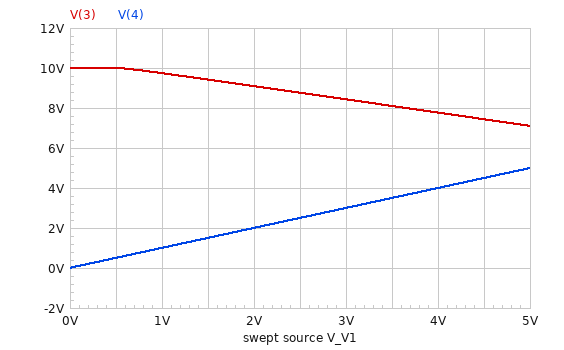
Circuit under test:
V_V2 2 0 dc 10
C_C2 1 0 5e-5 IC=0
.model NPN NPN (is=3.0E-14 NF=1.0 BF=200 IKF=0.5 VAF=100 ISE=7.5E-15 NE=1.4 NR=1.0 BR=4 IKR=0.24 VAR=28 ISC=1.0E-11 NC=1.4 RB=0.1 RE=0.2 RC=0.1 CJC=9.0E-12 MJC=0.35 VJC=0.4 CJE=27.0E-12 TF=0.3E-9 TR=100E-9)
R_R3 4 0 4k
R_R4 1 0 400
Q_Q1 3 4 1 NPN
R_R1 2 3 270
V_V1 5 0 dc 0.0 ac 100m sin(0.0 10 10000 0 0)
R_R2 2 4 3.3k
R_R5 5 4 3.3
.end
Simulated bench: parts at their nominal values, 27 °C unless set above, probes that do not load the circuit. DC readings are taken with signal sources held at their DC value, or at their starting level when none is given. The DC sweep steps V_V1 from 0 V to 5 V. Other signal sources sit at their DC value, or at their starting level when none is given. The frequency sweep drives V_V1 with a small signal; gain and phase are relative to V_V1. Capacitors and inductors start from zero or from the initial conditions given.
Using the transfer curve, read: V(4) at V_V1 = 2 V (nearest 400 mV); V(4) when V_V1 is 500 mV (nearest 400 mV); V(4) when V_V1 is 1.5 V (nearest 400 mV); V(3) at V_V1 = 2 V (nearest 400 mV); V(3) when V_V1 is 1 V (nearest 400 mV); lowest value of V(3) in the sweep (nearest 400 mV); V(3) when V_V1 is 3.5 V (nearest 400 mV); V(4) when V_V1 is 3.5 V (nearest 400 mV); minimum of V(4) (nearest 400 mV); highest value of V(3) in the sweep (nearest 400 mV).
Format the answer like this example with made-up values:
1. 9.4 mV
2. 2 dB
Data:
1. 2.0 V
2. 400 mV
3. 1.6 V
4. 9.2 V
5. 9.6 V
6. 7.2 V
7. 8.0 V
8. 3.6 V
9. 0 V
10. 10.0 V
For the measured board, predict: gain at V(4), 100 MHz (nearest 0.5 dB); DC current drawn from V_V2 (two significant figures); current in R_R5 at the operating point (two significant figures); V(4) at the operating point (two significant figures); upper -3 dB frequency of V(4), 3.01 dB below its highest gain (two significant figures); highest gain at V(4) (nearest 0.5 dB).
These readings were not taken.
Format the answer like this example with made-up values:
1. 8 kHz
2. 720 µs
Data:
1. 0 dB
2. 3.0 mA
3. 3.0 mA
4. 10 mV
5. 1.6 GHz
6. 0 dB
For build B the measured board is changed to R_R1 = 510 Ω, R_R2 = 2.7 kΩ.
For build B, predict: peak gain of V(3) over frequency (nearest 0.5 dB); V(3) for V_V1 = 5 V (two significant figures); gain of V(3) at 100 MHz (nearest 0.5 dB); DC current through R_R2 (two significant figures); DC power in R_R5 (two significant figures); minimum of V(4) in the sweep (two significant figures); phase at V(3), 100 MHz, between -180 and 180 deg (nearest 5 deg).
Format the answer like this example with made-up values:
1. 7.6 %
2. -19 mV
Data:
1. -0.5 dB
2. 4.5 V
3. -3.5 dB
4. 3.7 mA
5. 45 µW
6. 12 mV
7. 45 deg
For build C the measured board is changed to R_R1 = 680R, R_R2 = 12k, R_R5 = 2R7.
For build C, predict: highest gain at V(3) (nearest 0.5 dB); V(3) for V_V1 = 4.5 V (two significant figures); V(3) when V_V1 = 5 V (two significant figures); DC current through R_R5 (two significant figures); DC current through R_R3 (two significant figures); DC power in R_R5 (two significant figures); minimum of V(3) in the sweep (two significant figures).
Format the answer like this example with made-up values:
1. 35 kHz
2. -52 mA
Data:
1. -0.5 dB
2. 3.9 V
3. 4.3 V
4. 830 µA
5. 560 nA
6. 1.9 µW
7. 3.8 V
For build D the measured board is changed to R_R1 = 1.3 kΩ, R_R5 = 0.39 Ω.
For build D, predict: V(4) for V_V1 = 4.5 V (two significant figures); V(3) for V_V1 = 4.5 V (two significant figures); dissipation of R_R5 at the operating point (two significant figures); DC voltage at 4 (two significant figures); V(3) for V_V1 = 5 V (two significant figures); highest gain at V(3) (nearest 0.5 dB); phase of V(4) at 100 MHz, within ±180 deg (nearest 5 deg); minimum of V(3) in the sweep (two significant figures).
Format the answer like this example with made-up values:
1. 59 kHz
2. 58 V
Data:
1. 4.5 V
2. 3.8 V
3. 3.6 µW
4. 1.2 mV
5. 4.3 V
6. 0 dB
7. 0 deg
8. 2.5 V
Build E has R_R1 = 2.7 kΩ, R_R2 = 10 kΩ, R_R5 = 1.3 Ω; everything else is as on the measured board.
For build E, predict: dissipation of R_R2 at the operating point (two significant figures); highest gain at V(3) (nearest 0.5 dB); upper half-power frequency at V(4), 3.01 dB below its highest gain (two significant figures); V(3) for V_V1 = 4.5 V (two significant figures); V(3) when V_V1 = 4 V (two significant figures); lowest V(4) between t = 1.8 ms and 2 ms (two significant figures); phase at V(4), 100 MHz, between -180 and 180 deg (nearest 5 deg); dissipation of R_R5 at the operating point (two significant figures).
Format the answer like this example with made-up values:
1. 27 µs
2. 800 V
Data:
1. 10 mW
2. 0 dB
3. 3.8 GHz
4. 3.8 V
5. 3.3 V
6. -10 V
7. 0 deg
8. 1.3 µW
